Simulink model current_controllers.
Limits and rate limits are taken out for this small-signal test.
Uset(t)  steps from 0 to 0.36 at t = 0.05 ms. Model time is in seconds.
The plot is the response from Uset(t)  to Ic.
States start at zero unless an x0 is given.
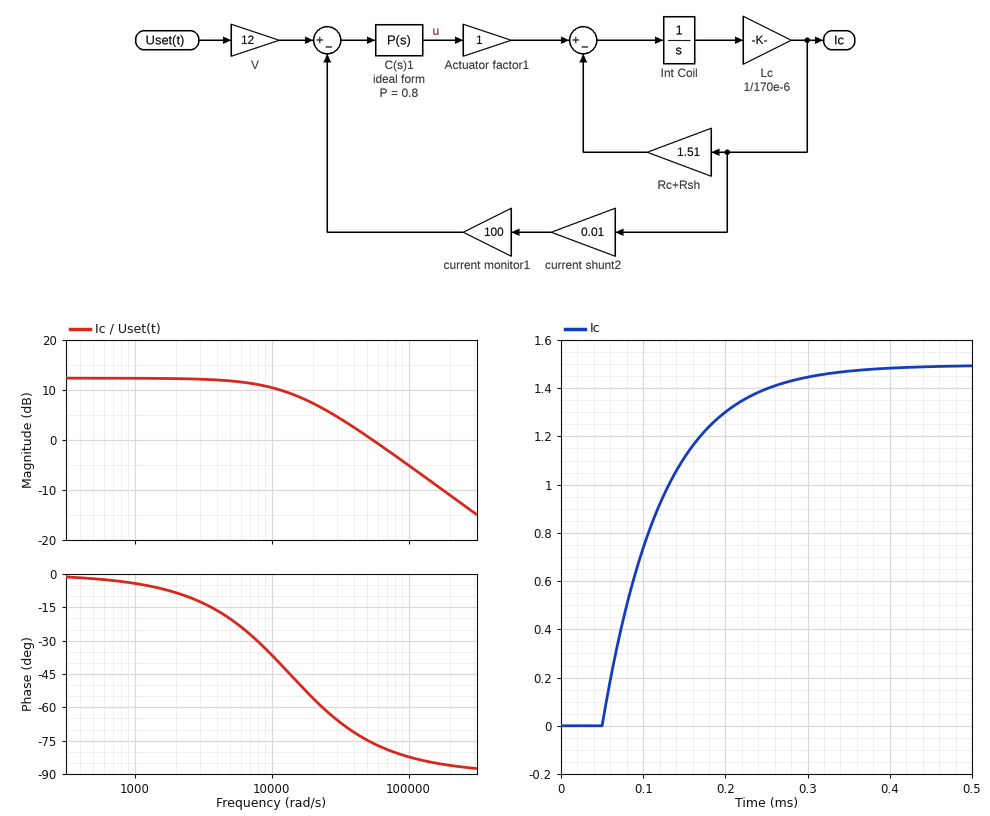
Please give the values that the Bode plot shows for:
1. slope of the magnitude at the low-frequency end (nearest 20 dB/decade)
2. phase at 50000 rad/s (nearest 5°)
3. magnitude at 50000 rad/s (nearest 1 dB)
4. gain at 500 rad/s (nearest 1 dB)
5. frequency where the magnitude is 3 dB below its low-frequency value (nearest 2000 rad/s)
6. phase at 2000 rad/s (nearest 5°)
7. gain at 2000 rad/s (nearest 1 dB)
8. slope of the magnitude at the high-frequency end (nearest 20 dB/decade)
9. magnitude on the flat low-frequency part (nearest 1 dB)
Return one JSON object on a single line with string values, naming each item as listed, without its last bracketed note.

{"slope of the magnitude at the low-frequency end": "0 dB/decade", "phase at 50000 rad/s": "-75°", "magnitude at 50000 rad/s": "1 dB", "gain at 500 rad/s": "12 dB", "frequency where the magnitude is 3 dB below its low-frequency value": "14000 rad/s", "phase at 2000 rad/s": "-10°", "gain at 2000 rad/s": "12 dB", "slope of the magnitude at the high-frequency end": "-20 dB/decade", "magnitude on the flat low-frequency part": "12 dB"}
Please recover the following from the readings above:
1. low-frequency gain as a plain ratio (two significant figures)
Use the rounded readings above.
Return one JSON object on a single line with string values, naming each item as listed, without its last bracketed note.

{"low-frequency gain as a plain ratio": "4.0"}
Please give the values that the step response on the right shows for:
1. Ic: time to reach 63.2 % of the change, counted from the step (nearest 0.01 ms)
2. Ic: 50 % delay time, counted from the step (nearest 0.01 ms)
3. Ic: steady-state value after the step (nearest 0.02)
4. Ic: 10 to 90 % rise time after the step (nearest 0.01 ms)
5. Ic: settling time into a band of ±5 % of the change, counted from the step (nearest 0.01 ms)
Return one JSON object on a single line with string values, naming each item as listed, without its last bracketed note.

{"Ic: time to reach 63.2 % of the change, counted from the step": "0.07 ms", "Ic: 50 % delay time, counted from the step": "0.05 ms", "Ic: steady-state value after the step": "1.50", "Ic: 10 to 90 % rise time after the step": "0.16 ms", "Ic: settling time into a band of ±5 % of the change, counted from the step": "0.22 ms"}
